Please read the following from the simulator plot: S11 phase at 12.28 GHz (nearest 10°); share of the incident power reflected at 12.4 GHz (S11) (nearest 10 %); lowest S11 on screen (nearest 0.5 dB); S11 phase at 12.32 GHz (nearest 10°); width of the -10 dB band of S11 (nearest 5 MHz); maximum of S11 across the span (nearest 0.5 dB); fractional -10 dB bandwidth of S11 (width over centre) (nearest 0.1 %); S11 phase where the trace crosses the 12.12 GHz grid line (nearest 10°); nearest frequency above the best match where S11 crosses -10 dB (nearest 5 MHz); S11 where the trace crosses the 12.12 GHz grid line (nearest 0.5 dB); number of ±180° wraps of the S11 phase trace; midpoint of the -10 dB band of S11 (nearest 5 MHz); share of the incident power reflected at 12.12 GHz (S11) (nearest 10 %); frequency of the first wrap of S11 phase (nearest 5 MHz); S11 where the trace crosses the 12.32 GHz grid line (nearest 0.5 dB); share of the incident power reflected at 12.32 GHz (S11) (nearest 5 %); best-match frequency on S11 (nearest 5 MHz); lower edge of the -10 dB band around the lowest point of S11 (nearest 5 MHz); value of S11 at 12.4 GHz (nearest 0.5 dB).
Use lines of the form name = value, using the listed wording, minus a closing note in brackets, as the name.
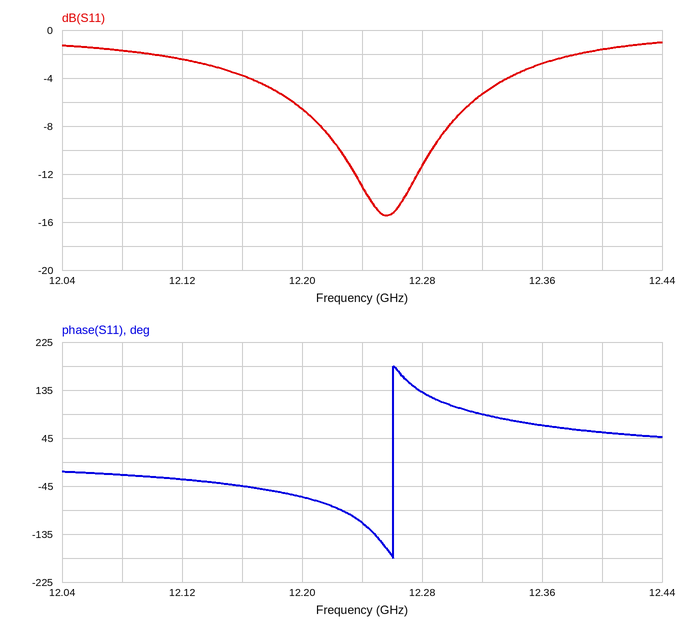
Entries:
S11 phase at 12.28 GHz = 130°
share of the incident power reflected at 12.4 GHz (S11) = 70 %
lowest S11 on screen = -15.5 dB
S11 phase at 12.32 GHz = 90°
width of the -10 dB band of S11 = 60 MHz
maximum of S11 across the span = -1.0 dB
fractional -10 dB bandwidth of S11 (width over centre) = 0.5 %
S11 phase where the trace crosses the 12.12 GHz grid line = -30°
nearest frequency above the best match where S11 crosses -10 dB = 12.285 GHz
S11 where the trace crosses the 12.12 GHz grid line = -2.5 dB
number of ±180° wraps of the S11 phase trace = 1
midpoint of the -10 dB band of S11 = 12.255 GHz
share of the incident power reflected at 12.12 GHz (S11) = 60 %
frequency of the first wrap of S11 phase = 12.260 GHz
S11 where the trace crosses the 12.32 GHz grid line = -5.5 dB
share of the incident power reflected at 12.32 GHz (S11) = 30 %
best-match frequency on S11 = 12.255 GHz
lower edge of the -10 dB band around the lowest point of S11 = 12.225 GHz
value of S11 at 12.4 GHz = -1.5 dB
